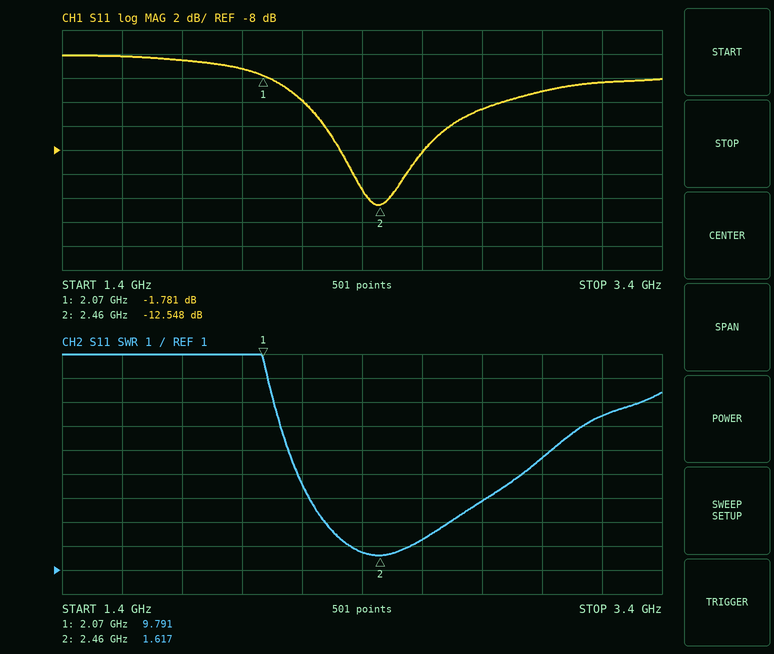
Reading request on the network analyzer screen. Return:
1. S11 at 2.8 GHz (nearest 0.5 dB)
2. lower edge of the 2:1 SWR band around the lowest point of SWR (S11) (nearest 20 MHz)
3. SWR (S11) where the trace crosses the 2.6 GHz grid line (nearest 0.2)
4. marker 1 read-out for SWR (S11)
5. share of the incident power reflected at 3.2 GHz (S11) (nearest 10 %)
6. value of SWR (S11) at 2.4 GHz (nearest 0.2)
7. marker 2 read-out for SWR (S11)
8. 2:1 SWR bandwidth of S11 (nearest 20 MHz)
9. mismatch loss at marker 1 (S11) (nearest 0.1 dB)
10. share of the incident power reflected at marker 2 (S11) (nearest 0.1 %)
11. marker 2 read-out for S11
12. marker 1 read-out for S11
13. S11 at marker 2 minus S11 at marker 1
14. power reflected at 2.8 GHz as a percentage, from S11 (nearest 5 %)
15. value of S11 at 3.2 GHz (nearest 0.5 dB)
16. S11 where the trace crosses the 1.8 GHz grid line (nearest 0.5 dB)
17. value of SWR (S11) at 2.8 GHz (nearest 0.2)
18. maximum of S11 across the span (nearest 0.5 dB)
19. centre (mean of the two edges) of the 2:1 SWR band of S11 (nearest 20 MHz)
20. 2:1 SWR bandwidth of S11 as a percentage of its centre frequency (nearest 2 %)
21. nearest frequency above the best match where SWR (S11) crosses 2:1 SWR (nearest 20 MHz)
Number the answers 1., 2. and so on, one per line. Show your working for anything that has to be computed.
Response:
1. -4.5 dB
2. 2.36 GHz
3. 2.2
4. 9.791
5. 10^(-2.5/10) ≈ 56.2 %, so 60 % to the nearest 10 %
6. 1.8
7. 1.617
8. 2.56 GHz − 2.36 GHz = 200 MHz
9. −10 log10(1 − 10^(-1.781/10)) ≈ 4.7 dB
10. 10^(-12.548/10) ≈ 5.6 %
11. -12.548 dB
12. -1.781 dB
13. -12.548 − (-1.781) = -10.767 dB
14. 10^(-4.5/10) ≈ 35 %
15. -2.5 dB
16. -0.5 dB
17. 3.8
18. 0.0 dB
19. 2.46 GHz
20. 200 MHz / 2.46 GHz ≈ 8 %
21. 2.56 GHz
